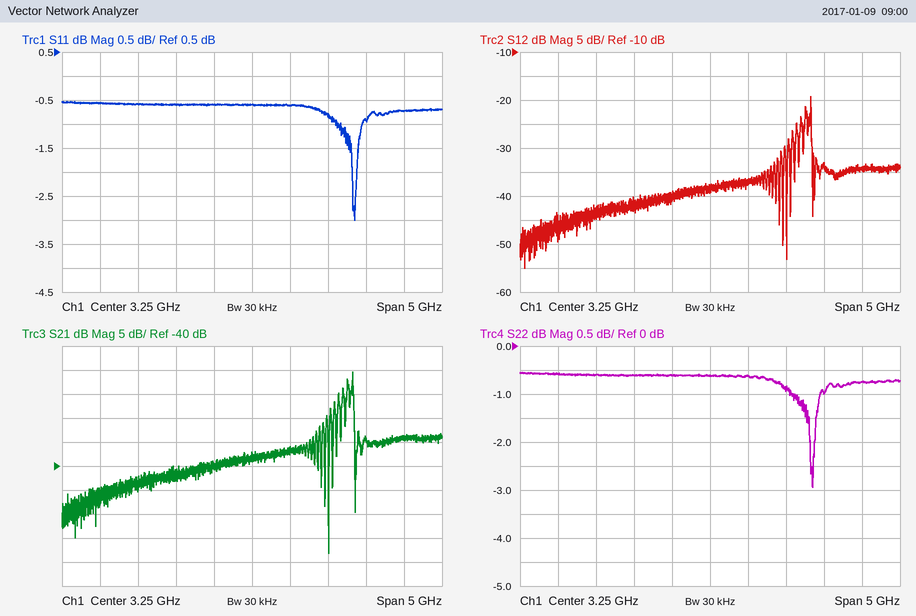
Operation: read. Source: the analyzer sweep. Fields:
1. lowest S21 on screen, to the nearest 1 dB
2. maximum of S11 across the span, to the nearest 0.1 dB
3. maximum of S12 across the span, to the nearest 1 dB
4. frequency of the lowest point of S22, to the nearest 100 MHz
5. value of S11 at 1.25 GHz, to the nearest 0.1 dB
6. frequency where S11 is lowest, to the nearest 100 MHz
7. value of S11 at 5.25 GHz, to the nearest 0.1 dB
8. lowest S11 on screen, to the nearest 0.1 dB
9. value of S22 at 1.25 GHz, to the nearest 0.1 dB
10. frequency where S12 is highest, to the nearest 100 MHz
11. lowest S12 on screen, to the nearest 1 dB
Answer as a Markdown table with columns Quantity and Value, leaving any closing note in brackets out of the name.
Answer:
| Quantity | Value |
|---|---|
| lowest S21 on screen, to the nearest 1 dB | -58 dB |
| maximum of S11 across the span, to the nearest 0.1 dB | -0.5 dB |
| maximum of S12 across the span, to the nearest 1 dB | -19 dB |
| frequency of the lowest point of S22, to the nearest 100 MHz | 4.6 GHz |
| value of S11 at 1.25 GHz, to the nearest 0.1 dB | -0.6 dB |
| frequency where S11 is lowest, to the nearest 100 MHz | 4.6 GHz |
| value of S11 at 5.25 GHz, to the nearest 0.1 dB | -0.7 dB |
| lowest S11 on screen, to the nearest 0.1 dB | -3.0 dB |
| value of S22 at 1.25 GHz, to the nearest 0.1 dB | -0.6 dB |
| frequency where S12 is highest, to the nearest 100 MHz | 4.6 GHz |
| lowest S12 on screen, to the nearest 1 dB | -55 dB |
